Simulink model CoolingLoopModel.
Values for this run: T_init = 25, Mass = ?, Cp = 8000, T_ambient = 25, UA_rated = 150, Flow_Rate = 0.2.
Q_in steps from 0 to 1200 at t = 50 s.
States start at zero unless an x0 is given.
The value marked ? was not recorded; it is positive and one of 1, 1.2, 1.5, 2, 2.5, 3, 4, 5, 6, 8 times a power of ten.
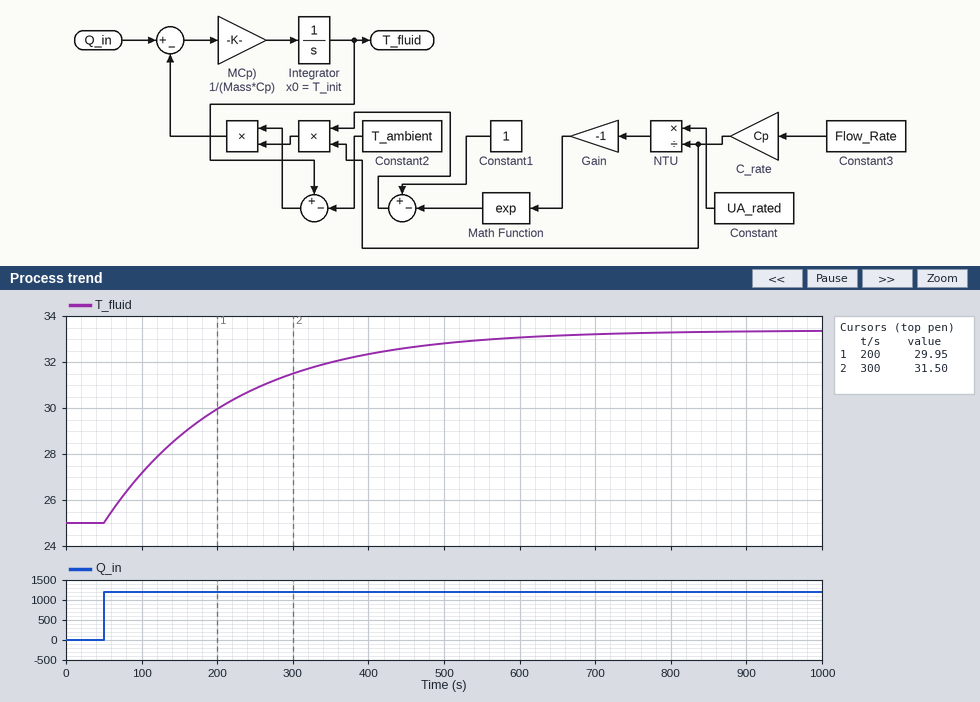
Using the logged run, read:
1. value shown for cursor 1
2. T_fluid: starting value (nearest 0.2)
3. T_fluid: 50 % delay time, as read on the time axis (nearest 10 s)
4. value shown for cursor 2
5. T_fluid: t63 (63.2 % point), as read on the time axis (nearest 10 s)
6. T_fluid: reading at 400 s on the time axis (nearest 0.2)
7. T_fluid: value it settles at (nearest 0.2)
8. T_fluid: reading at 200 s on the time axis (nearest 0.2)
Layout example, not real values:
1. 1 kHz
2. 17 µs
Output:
1. 29.95
2. 25.0
3. 170 s
4. 31.50
5. 220 s
6. 32.4
7. 33.4
8. 30.0
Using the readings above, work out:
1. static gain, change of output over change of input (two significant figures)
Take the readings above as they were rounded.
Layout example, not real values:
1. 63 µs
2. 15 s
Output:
1. 0.0070
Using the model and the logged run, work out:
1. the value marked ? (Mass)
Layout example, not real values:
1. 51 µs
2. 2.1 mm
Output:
1. 3
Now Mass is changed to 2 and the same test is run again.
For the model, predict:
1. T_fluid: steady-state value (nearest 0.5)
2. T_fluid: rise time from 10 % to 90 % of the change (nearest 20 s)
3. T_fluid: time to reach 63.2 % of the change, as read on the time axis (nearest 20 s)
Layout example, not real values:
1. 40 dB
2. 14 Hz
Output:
1. 33.5
2. 240 s
3. 160 s
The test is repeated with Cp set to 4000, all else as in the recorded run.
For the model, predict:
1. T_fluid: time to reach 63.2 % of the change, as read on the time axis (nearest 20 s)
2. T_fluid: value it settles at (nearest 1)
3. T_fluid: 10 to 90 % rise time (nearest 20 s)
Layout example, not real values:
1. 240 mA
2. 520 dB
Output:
1. 140 s
2. 34
3. 200 s
